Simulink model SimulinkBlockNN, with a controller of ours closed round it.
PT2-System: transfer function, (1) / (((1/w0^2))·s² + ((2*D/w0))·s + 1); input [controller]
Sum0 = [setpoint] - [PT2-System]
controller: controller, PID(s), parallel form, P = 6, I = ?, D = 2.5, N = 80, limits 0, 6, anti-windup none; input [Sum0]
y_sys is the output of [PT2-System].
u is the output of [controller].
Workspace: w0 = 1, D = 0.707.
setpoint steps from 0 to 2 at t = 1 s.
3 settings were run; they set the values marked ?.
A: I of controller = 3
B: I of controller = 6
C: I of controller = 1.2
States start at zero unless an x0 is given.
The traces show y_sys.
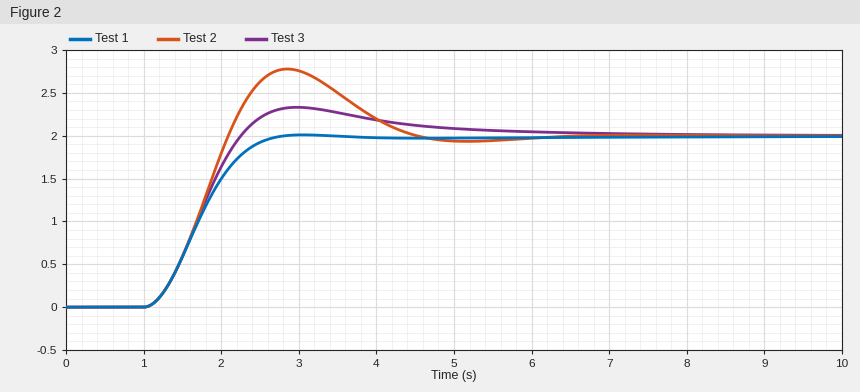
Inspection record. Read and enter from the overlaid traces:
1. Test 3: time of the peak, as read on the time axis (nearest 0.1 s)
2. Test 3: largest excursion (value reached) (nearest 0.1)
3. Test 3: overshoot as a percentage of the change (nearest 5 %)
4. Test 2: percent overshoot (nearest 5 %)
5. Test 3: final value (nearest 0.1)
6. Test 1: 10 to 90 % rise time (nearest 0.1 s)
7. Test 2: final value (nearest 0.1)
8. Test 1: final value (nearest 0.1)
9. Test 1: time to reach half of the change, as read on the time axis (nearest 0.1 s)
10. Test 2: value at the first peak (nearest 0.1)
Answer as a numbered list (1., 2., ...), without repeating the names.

1. 3.0 s
2. 2.3
3. 15 %
4. 40 %
5. 2.0
6. 1.0 s
7. 2.0
8. 2.0
9. 1.7 s
10. 2.8
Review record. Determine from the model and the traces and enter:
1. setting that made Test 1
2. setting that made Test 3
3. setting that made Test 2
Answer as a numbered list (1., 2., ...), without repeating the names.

1. C
2. A
3. B
